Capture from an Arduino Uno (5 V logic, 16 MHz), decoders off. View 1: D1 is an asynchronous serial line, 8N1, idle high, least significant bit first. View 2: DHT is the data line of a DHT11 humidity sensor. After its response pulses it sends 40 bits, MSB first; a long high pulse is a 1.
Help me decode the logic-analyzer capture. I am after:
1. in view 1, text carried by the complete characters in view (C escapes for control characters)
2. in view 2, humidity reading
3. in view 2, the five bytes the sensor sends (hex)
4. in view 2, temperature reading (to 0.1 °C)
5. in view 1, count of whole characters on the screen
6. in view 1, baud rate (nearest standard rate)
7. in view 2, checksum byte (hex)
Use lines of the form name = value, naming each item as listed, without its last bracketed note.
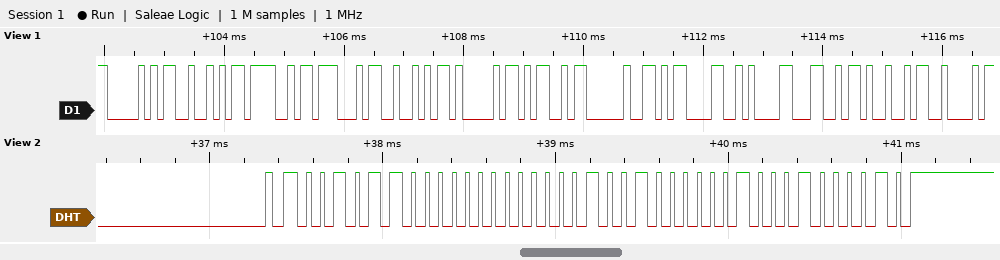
in view 1, text carried by the complete characters in view = "PROGRAM \r\nLIB"
in view 2, humidity reading = 44 %
in view 2, the five bytes the sensor sends = 2C 00 12 04 42
in view 2, temperature reading = 18.4 °C
in view 1, count of whole characters on the screen = 13
in view 1, baud rate = 9600 baud
in view 2, checksum byte = 0x42
